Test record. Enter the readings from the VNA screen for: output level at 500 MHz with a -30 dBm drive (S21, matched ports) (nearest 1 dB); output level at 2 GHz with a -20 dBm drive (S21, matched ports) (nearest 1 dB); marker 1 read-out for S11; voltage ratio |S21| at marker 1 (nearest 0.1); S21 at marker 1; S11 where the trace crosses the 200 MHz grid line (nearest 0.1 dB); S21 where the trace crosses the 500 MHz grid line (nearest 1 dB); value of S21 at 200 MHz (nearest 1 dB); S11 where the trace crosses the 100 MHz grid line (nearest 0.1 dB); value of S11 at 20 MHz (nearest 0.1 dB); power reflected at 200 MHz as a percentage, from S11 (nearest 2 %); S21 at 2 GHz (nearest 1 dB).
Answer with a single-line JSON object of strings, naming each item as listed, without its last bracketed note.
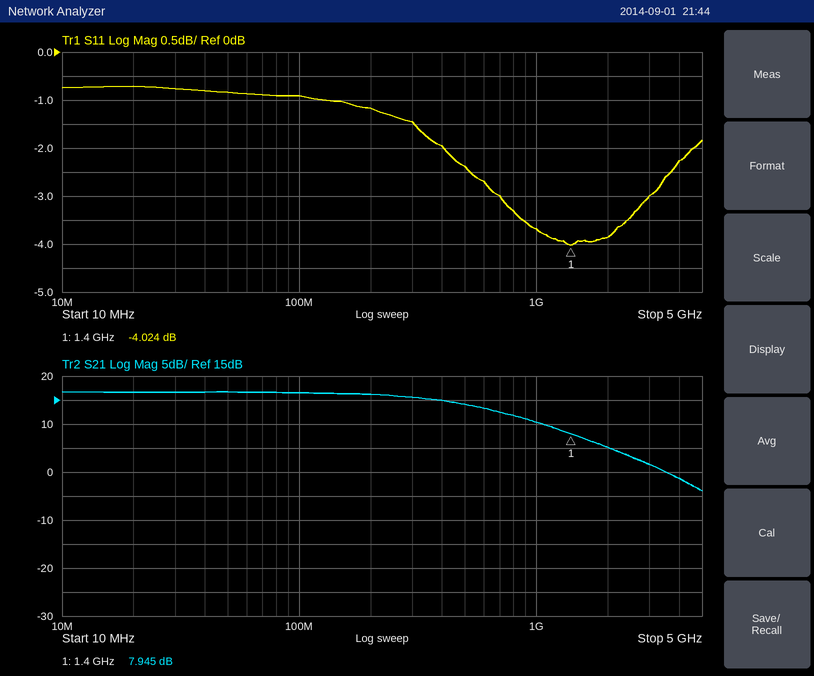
{"output level at 500 MHz with a -30 dBm drive (S21, matched ports)": "-16 dBm", "output level at 2 GHz with a -20 dBm drive (S21, matched ports)": "-15 dBm", "marker 1 read-out for S11": "-4.024 dB", "voltage ratio |S21| at marker 1": "2.5", "S21 at marker 1": "7.945 dB", "S11 where the trace crosses the 200 MHz grid line": "-1.2 dB", "S21 where the trace crosses the 500 MHz grid line": "14 dB", "value of S21 at 200 MHz": "16 dB", "S11 where the trace crosses the 100 MHz grid line": "-0.9 dB", "value of S11 at 20 MHz": "-0.7 dB", "power reflected at 200 MHz as a percentage, from S11": "76 %", "S21 at 2 GHz": "5 dB"}
